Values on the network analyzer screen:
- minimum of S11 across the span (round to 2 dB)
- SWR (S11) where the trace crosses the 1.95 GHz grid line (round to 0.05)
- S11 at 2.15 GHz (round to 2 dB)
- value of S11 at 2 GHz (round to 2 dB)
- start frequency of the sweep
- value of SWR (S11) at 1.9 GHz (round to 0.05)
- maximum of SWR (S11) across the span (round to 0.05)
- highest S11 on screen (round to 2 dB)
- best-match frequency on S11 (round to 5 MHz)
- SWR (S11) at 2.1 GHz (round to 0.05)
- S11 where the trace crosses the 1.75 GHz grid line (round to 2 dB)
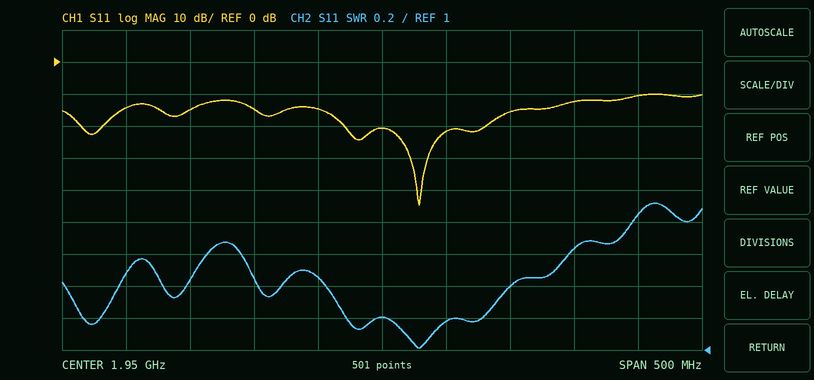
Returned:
-44 dB
1.20
-10 dB
-22 dB
1.7 GHz
1.45
1.90
-10 dB
1.980 GHz
1.65
-14 dB
